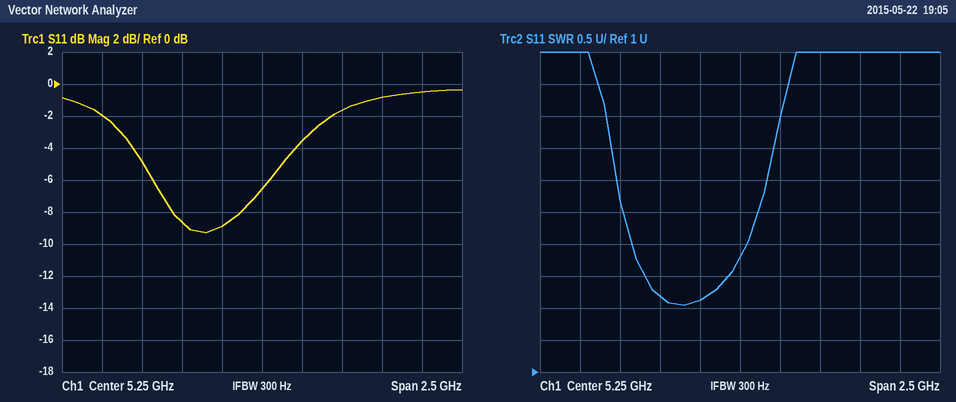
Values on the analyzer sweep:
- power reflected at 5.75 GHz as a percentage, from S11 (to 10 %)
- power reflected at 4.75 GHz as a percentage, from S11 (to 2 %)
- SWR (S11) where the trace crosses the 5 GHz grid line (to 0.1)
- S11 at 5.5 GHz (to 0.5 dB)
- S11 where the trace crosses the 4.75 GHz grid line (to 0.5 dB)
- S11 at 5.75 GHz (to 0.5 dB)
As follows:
70 %
14 %
2.1
-3.5 dB
-8.5 dB
-1.5 dB
